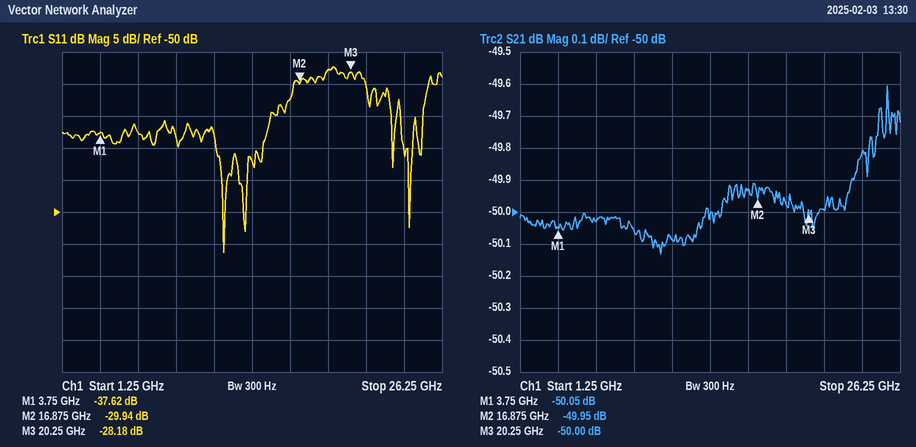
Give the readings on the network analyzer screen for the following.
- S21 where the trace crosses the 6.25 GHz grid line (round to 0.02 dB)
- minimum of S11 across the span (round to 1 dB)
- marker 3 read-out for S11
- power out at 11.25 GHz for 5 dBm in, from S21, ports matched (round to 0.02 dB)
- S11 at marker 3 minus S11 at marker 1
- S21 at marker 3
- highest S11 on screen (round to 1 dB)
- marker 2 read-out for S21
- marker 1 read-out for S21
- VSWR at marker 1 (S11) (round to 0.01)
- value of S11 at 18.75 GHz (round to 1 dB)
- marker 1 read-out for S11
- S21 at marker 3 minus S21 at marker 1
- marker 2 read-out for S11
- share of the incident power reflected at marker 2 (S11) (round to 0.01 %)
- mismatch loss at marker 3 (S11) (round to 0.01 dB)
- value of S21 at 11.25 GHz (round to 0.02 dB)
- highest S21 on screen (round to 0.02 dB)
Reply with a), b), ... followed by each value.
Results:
a) -50.02 dB
b) -56 dB
c) -28.18 dB
d) -45.08 dBm
e) 9.44 dB
f) -50.00 dB
g) -27 dB
h) -49.95 dB
i) -50.05 dB
j) 1.03
k) -28 dB
l) -37.62 dB
m) 0.05 dB
n) -29.94 dB
o) 0.10 %
p) 0.01 dB
q) -50.08 dB
r) -49.60 dB
